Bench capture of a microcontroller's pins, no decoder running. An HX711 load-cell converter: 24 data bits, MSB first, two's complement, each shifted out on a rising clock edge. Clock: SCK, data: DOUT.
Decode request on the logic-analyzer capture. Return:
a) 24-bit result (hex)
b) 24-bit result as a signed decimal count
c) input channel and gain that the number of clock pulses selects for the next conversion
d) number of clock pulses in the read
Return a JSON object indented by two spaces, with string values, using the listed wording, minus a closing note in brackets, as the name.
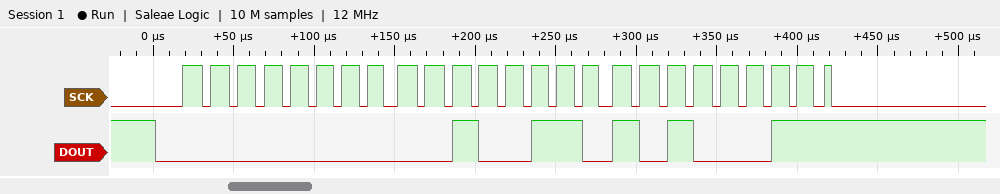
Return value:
{
  "24-bit result": "0x0026A3",
  "24-bit result as a signed decimal count": "9891",
  "input channel and gain that the number of clock pulses selects for the next conversion": "channel A, gain 128",
  "number of clock pulses in the read": "25"
}
